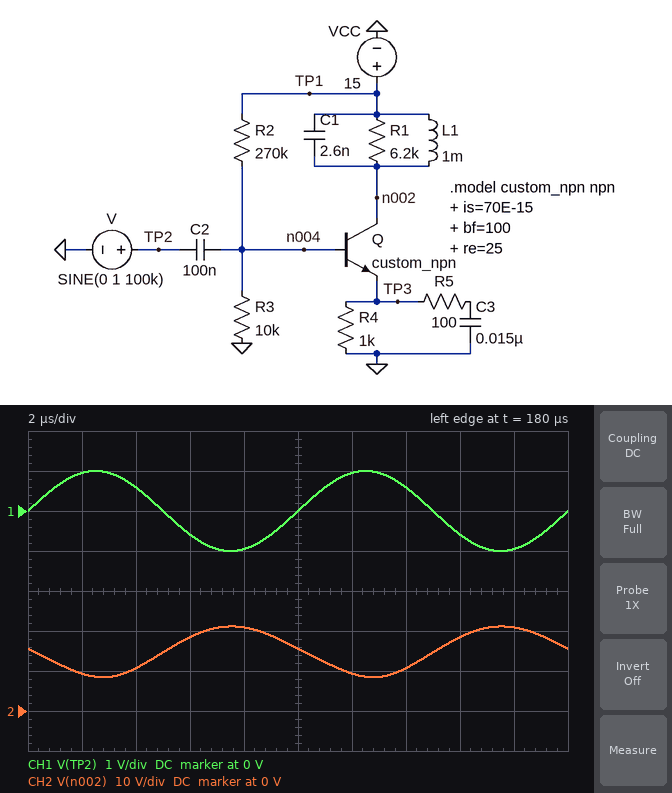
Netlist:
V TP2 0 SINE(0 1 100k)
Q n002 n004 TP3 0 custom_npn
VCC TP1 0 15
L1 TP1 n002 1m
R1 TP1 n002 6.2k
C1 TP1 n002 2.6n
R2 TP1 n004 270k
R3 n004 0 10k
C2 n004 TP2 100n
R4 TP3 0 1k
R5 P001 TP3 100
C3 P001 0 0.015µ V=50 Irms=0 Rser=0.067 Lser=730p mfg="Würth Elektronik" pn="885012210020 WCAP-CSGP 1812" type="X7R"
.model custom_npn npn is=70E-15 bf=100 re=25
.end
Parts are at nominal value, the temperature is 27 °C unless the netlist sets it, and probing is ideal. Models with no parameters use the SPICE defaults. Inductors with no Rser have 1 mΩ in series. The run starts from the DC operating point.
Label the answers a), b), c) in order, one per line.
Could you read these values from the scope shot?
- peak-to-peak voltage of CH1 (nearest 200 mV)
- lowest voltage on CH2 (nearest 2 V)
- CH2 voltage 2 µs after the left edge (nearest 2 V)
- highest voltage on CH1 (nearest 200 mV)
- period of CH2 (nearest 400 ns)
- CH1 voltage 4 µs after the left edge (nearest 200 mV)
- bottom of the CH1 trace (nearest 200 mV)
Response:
a) 2.0 V
b) 8 V
c) 10 V
d) 1.0 V
e) 10.0 µs
f) 600 mV
g) -1.0 V
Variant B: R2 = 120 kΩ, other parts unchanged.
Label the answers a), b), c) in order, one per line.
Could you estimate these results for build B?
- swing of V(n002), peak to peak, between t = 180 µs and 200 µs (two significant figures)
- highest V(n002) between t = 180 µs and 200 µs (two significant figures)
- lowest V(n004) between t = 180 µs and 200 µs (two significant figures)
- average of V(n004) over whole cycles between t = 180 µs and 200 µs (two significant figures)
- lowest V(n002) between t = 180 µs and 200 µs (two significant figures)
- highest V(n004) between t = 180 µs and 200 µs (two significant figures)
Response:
a) 21 V
b) 25 V
c) 97 mV
d) 1.1 V
e) 4.2 V
f) 2.1 V
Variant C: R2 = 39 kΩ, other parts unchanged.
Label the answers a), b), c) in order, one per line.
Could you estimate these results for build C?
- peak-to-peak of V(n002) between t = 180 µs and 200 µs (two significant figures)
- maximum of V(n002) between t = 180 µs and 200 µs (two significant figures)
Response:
a) 25 V
b) 28 V
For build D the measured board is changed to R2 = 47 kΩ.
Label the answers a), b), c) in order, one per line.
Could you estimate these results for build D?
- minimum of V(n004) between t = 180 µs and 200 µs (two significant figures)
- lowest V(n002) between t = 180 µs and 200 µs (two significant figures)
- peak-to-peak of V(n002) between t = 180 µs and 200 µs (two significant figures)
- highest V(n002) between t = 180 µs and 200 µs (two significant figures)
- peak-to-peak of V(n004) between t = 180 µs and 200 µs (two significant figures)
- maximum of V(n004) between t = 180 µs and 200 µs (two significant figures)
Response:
a) 900 mV
b) 2.2 V
c) 25 V
d) 28 V
e) 2.0 V
f) 2.9 V
